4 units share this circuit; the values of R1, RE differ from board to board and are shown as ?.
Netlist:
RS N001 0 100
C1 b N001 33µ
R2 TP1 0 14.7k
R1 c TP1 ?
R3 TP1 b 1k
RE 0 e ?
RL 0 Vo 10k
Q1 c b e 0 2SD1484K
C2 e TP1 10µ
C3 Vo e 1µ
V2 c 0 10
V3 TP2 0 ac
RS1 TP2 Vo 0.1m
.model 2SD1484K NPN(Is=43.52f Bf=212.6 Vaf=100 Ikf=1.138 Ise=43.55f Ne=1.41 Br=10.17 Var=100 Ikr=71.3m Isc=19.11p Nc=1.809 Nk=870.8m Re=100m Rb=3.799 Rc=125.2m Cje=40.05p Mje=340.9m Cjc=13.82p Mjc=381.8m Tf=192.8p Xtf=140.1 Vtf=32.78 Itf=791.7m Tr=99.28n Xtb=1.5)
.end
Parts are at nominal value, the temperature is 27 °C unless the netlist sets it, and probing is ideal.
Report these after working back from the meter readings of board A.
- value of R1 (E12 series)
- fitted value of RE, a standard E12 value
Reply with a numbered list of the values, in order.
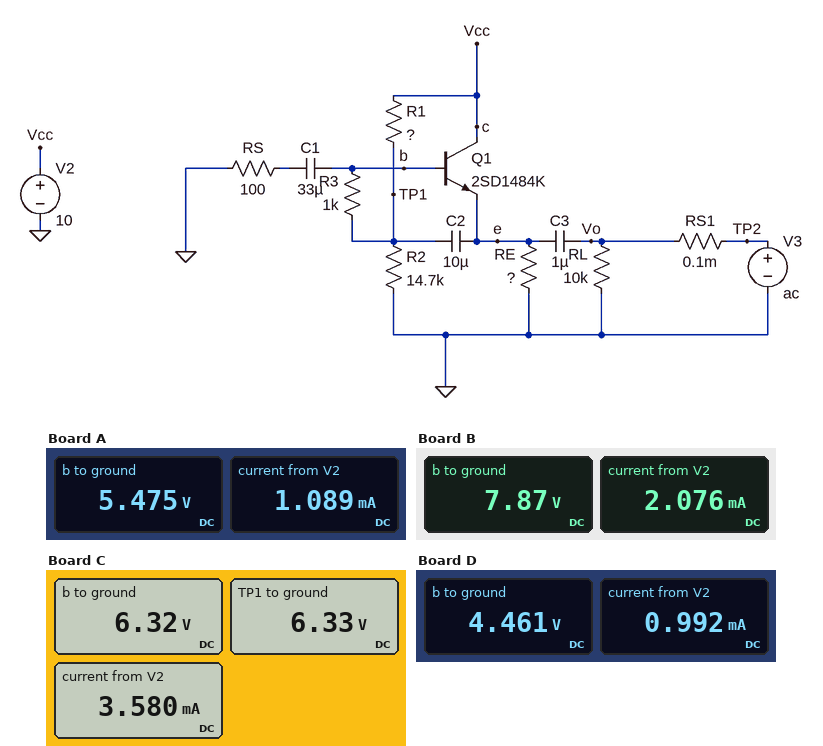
1. 12 kΩ
2. 6.8 kΩ
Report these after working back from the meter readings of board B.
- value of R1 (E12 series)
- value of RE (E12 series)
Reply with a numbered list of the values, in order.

1. 3.9 kΩ
2. 4.7 kΩ
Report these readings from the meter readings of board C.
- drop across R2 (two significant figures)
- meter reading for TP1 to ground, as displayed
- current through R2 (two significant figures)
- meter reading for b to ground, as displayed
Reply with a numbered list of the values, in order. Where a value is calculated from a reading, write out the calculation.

1. 6.33 V = 6.3 V
2. 6.33 V
3. (6.33 V) / 14.7 kΩ = 430 µA
4. 6.32 V
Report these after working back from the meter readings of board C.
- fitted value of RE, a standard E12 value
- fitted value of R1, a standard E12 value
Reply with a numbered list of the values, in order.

1. 1.8 kΩ
2. 8.2 kΩ
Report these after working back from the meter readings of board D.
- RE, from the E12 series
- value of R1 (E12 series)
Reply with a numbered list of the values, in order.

1. 5.6 kΩ
2. 18 kΩ
